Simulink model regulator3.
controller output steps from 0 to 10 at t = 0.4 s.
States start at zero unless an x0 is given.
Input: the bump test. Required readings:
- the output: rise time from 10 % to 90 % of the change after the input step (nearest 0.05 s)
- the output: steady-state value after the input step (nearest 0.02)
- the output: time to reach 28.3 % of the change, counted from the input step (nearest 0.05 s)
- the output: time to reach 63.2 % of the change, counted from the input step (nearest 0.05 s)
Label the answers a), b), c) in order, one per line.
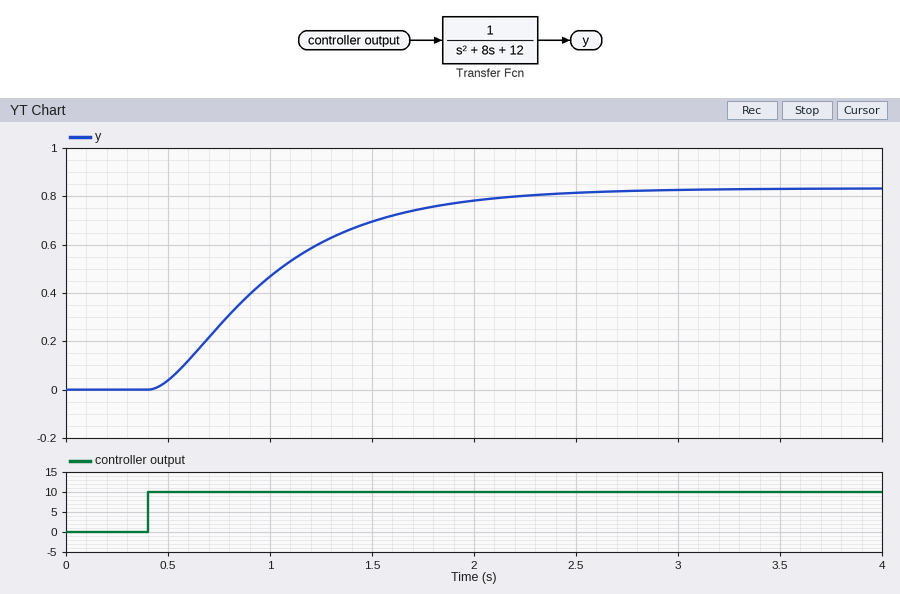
a) 1.20 s
b) 0.84
c) 0.30 s
d) 0.70 s
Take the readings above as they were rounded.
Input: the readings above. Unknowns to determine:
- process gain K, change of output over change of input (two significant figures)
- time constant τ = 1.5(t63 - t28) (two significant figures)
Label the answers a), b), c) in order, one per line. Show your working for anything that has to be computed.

a) (0.84 - 0) / 10 = 0.084
b) 1.5 × (0.7 - 0.3) = 0.60 s
